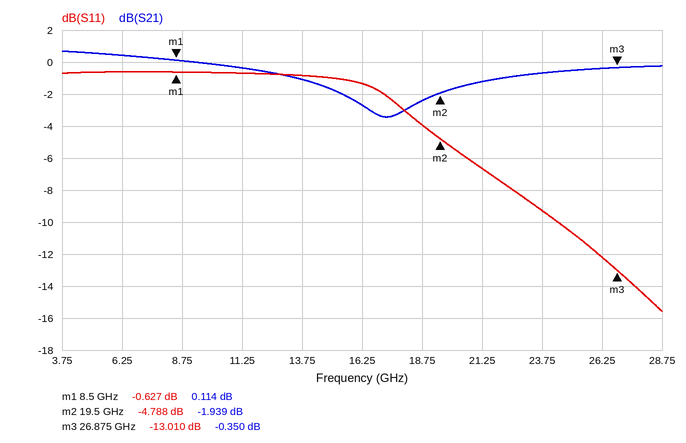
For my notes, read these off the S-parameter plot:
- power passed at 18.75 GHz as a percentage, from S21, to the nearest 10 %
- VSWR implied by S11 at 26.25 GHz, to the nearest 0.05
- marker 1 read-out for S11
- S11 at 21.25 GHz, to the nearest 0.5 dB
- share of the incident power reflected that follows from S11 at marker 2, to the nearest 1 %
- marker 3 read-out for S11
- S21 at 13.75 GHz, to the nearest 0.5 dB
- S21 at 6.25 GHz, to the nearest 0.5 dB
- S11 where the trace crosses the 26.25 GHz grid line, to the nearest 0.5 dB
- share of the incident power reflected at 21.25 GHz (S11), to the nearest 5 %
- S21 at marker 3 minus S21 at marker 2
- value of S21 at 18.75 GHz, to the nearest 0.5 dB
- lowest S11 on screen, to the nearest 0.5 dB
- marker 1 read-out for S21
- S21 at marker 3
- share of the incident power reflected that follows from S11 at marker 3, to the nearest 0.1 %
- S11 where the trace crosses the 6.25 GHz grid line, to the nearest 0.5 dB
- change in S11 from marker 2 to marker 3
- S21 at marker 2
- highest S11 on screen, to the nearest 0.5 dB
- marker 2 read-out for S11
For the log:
60 %
1.65
-0.627 dB
-6.5 dB
33 %
-13.010 dB
-1.0 dB
0.5 dB
-12.0 dB
20 %
1.589 dB
-2.5 dB
-15.5 dB
0.114 dB
-0.350 dB
5.0 %
-0.5 dB
-8.222 dB
-1.939 dB
-0.5 dB
-4.788 dB
